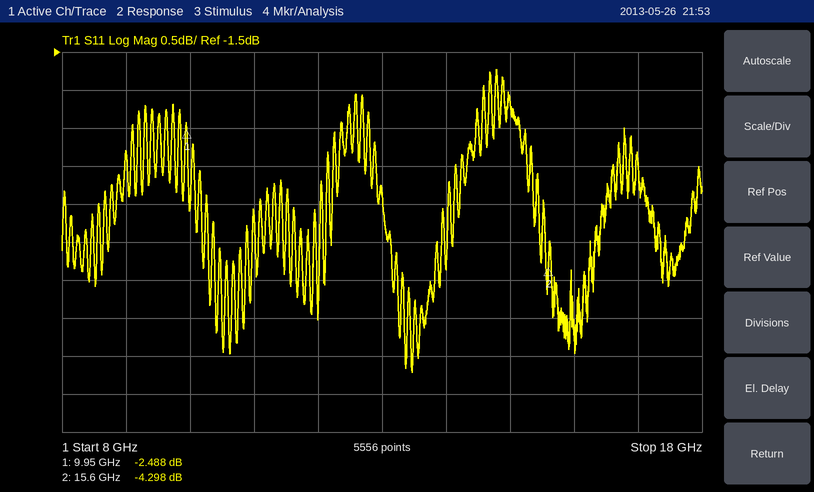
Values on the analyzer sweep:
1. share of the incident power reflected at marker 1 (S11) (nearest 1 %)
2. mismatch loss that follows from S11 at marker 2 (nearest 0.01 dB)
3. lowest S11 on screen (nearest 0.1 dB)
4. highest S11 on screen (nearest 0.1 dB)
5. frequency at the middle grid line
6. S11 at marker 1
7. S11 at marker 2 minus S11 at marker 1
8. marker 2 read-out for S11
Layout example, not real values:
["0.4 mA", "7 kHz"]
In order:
["56 %", "2.02 dB", "-5.7 dB", "-1.7 dB", "13 GHz", "-2.488 dB", "-1.810 dB", "-4.298 dB"]
